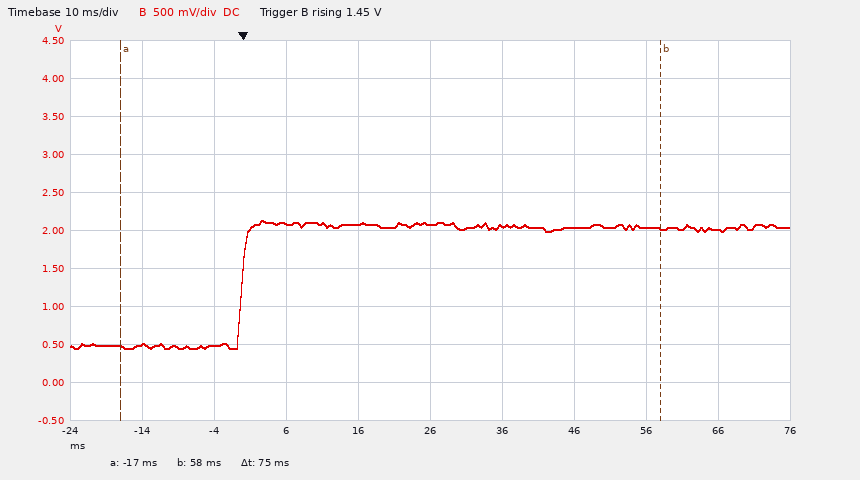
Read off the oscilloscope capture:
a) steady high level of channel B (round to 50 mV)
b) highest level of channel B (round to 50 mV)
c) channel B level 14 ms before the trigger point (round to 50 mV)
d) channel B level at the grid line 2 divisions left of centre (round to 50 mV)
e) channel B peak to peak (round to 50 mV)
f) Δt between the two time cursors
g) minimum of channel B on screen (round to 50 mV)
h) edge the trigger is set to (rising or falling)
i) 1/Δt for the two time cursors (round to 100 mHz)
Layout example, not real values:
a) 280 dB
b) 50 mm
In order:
a) 2.05 V
b) 2.15 V
c) 500 mV
d) 2.10 V
e) 1.70 V
f) 75 ms
g) 450 mV
h) rising
i) 13.3 Hz
